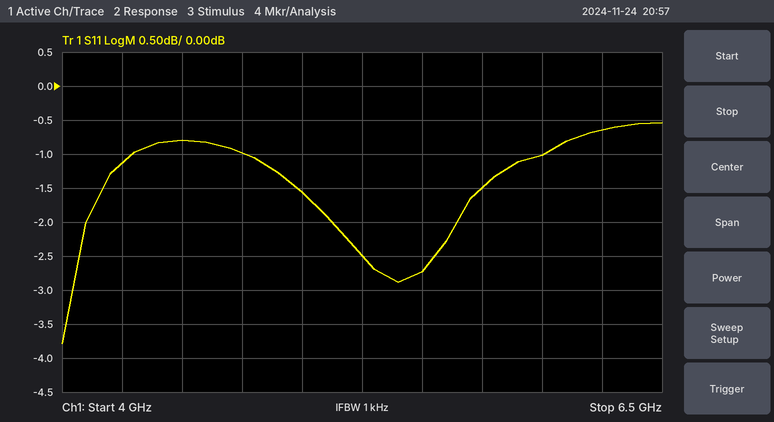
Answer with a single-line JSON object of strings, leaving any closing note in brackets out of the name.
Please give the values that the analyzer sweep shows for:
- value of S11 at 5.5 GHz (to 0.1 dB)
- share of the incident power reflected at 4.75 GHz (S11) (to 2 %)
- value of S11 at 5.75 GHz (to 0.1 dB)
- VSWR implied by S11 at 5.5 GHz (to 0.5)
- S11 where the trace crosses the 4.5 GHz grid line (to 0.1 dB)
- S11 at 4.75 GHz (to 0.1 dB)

{"value of S11 at 5.5 GHz": "-2.7 dB", "share of the incident power reflected at 4.75 GHz (S11)": "80 %", "value of S11 at 5.75 GHz": "-1.5 dB", "VSWR implied by S11 at 5.5 GHz": "6.5", "S11 where the trace crosses the 4.5 GHz grid line": "-0.8 dB", "S11 at 4.75 GHz": "-1.0 dB"}
